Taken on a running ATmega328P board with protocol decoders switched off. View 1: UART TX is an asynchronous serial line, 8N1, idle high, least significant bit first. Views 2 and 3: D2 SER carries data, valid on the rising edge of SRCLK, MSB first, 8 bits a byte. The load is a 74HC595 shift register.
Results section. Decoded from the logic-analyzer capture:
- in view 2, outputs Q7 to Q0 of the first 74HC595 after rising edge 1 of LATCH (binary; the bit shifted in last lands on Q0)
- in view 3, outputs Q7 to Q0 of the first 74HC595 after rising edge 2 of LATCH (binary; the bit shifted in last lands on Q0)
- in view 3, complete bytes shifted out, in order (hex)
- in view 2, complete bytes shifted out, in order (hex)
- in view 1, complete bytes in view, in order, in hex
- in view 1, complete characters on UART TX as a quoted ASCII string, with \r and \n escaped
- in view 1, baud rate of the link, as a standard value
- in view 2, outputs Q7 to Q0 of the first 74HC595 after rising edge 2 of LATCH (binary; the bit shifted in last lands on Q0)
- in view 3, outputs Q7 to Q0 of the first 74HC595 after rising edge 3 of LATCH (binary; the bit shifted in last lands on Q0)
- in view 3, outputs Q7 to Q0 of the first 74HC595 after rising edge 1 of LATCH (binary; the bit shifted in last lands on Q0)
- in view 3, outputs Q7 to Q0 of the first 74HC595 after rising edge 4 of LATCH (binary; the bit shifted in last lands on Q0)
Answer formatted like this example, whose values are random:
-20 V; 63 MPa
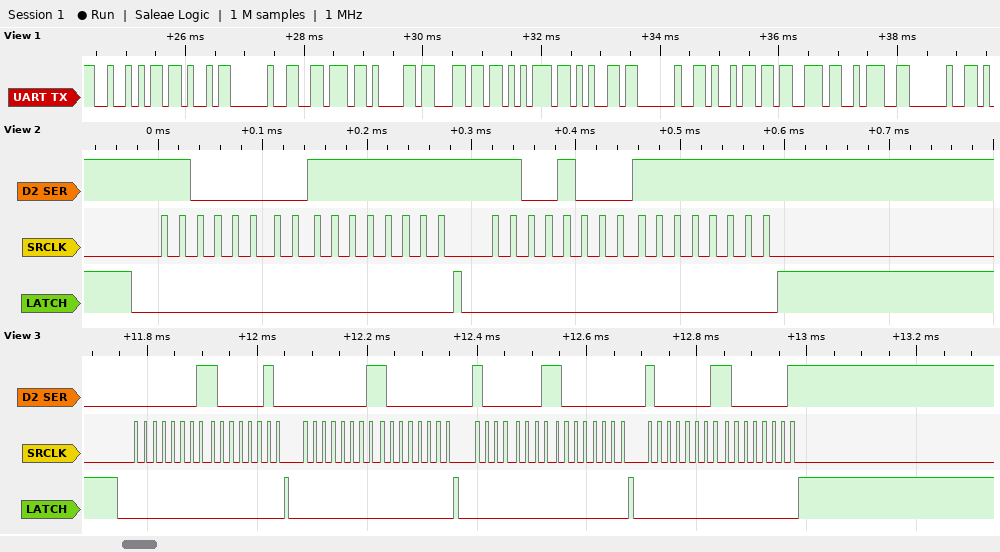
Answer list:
11111111; 10000000; 01 82 01 80 81 80 81 81; C0 FF C8 FF; 52 4B 20 76 61 6C 75 65 20 69 73 3A 20; "RK value is: "; 9600 baud; 11111111; 10000000; 10000010; 10000001
